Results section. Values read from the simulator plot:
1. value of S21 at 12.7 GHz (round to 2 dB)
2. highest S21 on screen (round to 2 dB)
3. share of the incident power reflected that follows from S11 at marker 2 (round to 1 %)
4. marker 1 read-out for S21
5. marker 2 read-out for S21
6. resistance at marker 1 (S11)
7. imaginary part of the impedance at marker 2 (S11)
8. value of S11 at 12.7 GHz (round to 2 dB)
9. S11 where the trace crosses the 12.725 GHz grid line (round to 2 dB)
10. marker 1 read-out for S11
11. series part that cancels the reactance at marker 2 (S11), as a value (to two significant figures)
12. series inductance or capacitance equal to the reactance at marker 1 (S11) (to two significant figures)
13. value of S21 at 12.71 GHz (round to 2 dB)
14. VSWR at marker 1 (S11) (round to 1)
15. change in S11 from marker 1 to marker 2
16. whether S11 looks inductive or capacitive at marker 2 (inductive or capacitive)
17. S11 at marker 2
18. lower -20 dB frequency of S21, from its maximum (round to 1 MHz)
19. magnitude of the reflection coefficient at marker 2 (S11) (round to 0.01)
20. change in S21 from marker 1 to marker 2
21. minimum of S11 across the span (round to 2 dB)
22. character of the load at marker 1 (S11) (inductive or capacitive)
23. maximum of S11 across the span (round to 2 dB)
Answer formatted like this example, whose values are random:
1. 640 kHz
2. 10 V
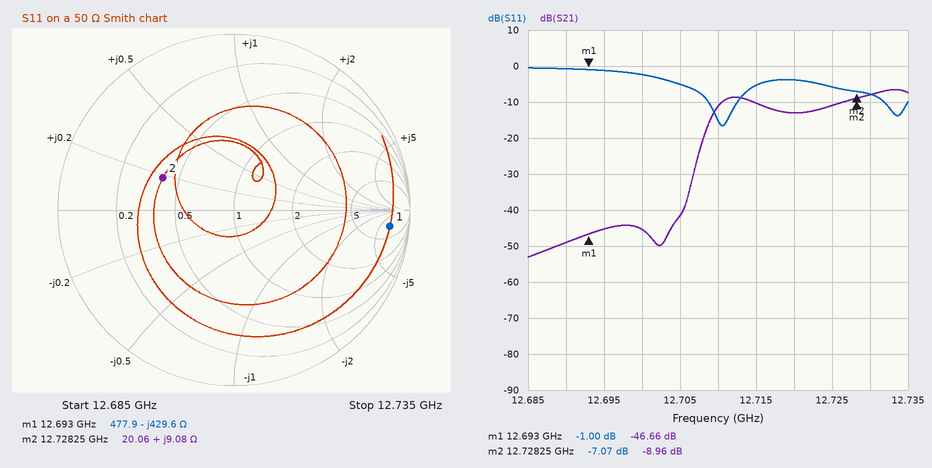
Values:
1. -46 dB
2. -6 dB
3. 20 %
4. -46.66 dB
5. -8.96 dB
6. 477.9 Ω
7. +9.08 Ω
8. -2 dB
9. -6 dB
10. -1.00 dB
11. 1.4 pF
12. 29 fF
13. -12 dB
14. 17
15. -6.07 dB
16. inductive
17. -7.07 dB
18. 12.707 GHz
19. 0.44
20. 37.70 dB
21. -16 dB
22. capacitive
23. 0 dB
